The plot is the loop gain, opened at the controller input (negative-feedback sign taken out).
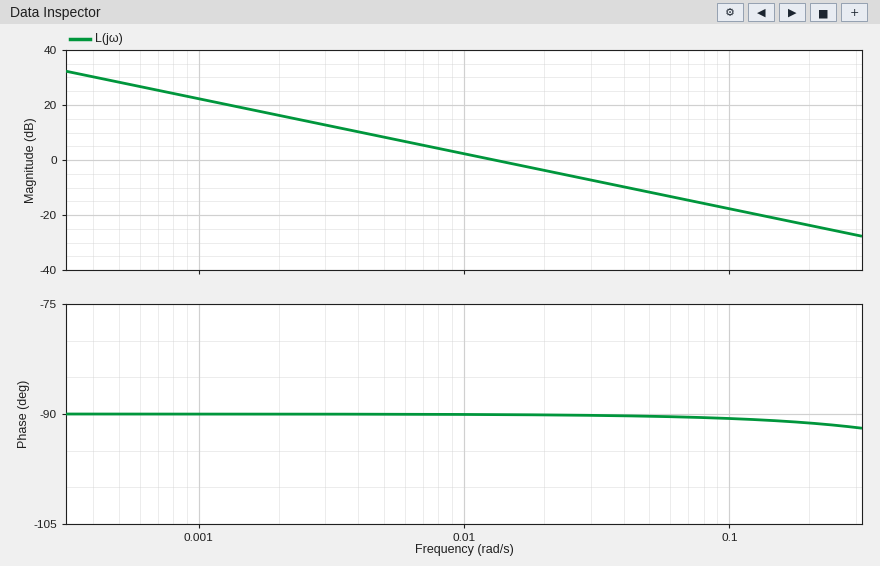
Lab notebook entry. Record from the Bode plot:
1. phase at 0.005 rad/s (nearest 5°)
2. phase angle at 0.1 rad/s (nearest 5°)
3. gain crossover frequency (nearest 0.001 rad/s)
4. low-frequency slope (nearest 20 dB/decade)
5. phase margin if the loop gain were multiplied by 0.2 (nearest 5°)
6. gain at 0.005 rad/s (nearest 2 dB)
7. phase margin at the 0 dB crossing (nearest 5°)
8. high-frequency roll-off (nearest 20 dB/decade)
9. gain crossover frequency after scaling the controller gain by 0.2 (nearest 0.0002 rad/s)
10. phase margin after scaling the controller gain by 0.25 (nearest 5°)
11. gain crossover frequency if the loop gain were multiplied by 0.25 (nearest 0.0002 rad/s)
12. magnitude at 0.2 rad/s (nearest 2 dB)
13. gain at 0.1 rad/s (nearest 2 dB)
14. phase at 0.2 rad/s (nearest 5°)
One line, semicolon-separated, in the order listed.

-90°; -90°; 0.013 rad/s; -20 dB/decade; 90°; 8 dB; 90°; -20 dB/decade; 0.0026 rad/s; 90°; 0.0032 rad/s; -24 dB; -18 dB; -90°
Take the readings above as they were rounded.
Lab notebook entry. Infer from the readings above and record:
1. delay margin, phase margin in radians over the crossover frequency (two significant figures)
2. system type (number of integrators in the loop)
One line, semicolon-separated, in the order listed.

120 s; 1
